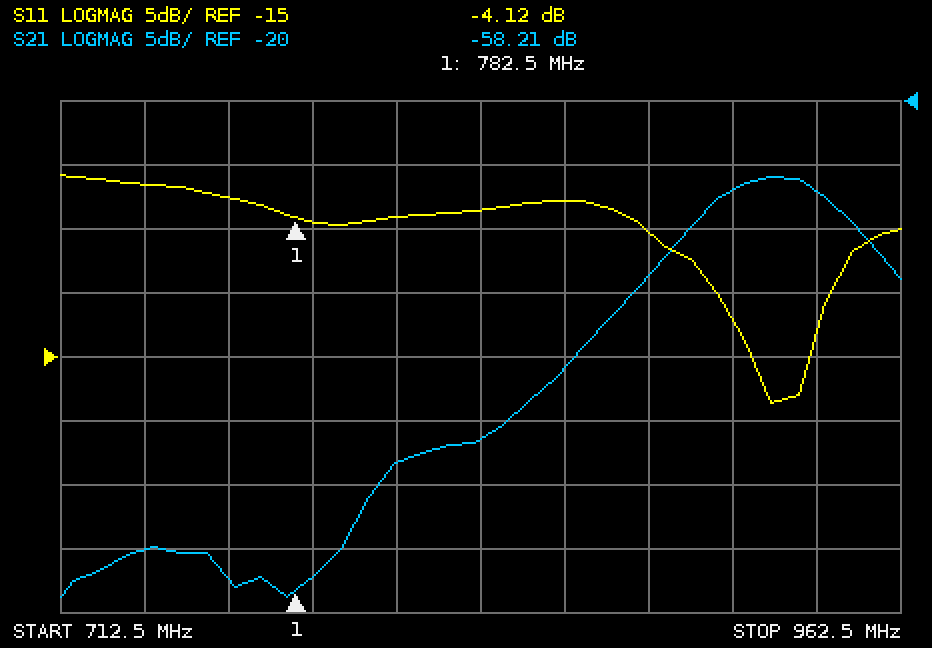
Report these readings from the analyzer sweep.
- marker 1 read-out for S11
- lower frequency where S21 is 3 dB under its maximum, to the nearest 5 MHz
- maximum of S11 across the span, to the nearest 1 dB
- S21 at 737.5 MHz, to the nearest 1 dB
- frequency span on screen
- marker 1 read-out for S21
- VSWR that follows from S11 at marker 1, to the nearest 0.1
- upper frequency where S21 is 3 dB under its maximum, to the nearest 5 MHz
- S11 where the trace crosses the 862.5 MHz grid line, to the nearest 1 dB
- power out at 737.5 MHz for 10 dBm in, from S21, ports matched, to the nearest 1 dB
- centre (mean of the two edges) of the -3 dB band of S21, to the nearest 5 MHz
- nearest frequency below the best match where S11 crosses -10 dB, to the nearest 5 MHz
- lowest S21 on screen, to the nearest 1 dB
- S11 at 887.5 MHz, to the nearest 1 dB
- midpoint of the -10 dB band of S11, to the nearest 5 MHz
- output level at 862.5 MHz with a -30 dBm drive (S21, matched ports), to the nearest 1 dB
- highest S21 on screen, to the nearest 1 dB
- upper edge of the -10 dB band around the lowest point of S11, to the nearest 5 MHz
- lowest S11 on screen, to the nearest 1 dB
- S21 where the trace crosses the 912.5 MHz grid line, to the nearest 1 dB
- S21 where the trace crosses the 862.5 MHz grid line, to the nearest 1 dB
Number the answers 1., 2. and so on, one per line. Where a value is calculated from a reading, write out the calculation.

1. -4.12 dB
2. 905 MHz
3. -1 dB
4. -55 dB
5. 250 MHz
6. -58.21 dB
7. (1 + 0.6223)/(1 − 0.6223) ≈ 4.3
8. 945 MHz
9. -3 dB
10. 10 dBm + (-55 dB) = -45 dBm
11. 925 MHz
12. 910 MHz
13. -59 dB
14. -5 dB
15. 925 MHz
16. -30 dBm + (-41 dB) = -71 dBm
17. -26 dB
18. 940 MHz
19. -19 dB
20. -27 dB
21. -41 dB
